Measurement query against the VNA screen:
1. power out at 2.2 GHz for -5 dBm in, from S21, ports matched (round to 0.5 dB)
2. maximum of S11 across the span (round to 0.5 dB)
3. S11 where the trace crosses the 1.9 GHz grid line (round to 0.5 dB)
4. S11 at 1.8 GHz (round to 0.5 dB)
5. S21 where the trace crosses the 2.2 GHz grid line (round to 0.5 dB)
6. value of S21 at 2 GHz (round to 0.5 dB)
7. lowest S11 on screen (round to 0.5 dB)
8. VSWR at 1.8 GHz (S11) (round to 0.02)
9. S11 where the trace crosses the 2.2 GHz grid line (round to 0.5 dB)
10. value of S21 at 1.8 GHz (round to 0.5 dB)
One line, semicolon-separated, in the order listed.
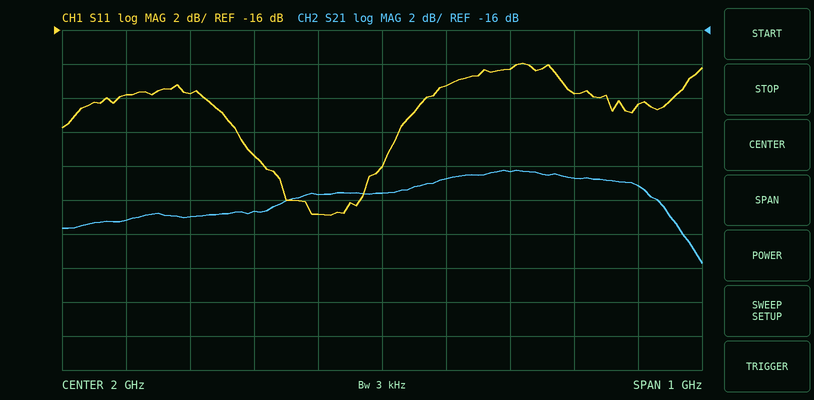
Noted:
-29.5 dBm; -18.0 dB; -27.0 dB; -23.5 dB; -24.5 dB; -25.5 dB; -27.0 dB; 1.14; -18.5 dB; -26.5 dB
